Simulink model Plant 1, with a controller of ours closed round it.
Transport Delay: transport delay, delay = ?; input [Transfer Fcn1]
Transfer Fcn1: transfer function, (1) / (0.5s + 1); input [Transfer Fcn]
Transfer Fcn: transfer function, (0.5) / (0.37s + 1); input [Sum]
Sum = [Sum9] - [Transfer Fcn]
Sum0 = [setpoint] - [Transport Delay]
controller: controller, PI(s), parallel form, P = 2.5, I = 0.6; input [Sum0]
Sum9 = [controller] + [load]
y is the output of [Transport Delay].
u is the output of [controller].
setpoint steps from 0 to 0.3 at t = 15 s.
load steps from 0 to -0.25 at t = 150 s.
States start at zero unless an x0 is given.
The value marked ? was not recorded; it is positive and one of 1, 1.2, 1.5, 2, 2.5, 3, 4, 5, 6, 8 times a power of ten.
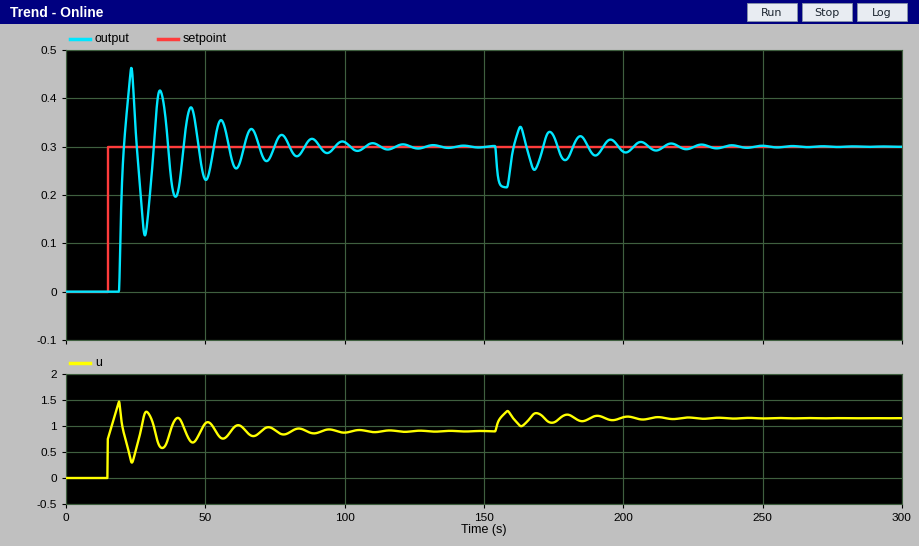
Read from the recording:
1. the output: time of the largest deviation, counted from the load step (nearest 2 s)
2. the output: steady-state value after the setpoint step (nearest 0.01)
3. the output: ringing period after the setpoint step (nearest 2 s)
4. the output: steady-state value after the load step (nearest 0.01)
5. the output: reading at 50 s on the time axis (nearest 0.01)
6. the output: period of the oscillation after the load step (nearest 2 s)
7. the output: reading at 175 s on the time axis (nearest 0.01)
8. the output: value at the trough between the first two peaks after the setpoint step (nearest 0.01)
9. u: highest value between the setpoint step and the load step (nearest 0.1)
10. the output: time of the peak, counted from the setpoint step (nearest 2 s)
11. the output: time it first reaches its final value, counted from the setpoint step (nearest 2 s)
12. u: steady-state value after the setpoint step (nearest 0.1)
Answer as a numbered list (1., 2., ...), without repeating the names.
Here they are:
1. 8 s
2. 0.30
3. 10 s
4. 0.30
5. 0.23
6. 10 s
7. 0.32
8. 0.12
9. 1.5
10. 8 s
11. 6 s
12. 0.9
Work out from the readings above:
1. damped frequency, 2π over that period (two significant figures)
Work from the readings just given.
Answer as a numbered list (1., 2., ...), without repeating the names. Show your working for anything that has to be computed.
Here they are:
1. 2π / 10 = 0.63 rad/s
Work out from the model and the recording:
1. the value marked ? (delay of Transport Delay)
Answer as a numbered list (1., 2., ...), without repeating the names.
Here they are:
1. 4
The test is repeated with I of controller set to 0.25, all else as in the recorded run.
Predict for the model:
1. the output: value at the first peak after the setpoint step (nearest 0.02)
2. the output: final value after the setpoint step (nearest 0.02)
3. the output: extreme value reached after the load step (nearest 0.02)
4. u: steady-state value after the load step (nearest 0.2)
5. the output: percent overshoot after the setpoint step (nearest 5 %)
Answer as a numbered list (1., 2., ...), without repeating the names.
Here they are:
1. 0.34
2. 0.30
3. 0.22
4. 1.2
5. 10 %
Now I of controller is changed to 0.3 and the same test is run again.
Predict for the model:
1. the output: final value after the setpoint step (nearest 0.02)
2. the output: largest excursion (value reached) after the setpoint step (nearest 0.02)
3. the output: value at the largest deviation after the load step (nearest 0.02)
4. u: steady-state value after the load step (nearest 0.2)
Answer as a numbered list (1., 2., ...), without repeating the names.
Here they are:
1. 0.30
2. 0.36
3. 0.22
4. 1.2
